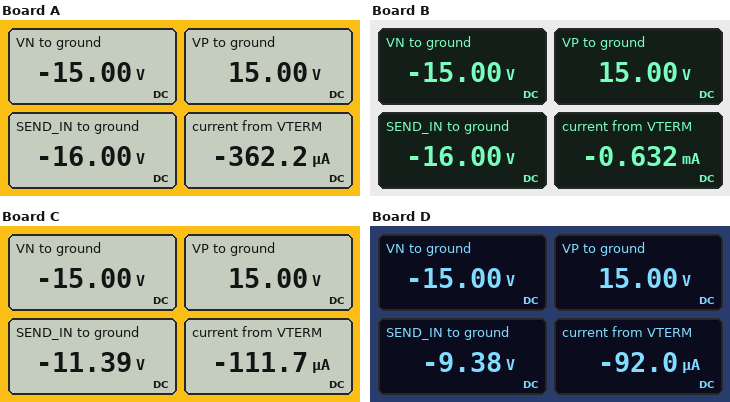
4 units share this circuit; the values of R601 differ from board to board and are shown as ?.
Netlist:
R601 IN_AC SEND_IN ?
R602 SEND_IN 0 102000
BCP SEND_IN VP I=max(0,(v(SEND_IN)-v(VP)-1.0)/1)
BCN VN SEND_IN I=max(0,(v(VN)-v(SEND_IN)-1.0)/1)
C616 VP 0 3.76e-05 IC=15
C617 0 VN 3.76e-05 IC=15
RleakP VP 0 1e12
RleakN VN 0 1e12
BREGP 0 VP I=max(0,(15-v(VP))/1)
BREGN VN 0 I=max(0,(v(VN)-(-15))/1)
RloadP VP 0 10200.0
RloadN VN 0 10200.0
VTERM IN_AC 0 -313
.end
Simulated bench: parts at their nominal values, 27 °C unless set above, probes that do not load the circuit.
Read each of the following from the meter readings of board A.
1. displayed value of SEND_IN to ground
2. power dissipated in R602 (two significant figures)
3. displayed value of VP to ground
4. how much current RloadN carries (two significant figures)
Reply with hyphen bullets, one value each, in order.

- -16.00 V
- 2.5 mW
- 15.00 V
- 1.5 mA
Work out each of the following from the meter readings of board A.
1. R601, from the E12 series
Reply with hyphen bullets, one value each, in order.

- 820 kΩ
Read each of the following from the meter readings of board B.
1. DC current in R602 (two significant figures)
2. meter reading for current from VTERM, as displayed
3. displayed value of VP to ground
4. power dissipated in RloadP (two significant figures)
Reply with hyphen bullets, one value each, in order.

- 160 µA
- -0.632 mA
- 15.00 V
- 22 mW
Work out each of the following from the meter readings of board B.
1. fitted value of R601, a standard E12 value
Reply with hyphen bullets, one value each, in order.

- 470 kΩ
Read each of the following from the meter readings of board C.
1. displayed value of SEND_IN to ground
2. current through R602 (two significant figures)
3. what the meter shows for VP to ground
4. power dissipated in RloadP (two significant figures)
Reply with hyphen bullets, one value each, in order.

- -11.39 V
- 110 µA
- 15.00 V
- 22 mW
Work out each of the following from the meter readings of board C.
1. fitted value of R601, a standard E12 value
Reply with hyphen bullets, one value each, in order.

- 2.7 MΩ
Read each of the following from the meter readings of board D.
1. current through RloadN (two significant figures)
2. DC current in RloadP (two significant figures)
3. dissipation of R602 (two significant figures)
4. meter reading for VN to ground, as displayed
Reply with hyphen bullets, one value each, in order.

- 1.5 mA
- 1.5 mA
- 860 µW
- -15.00 V
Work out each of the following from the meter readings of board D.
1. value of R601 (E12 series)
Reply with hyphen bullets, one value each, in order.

- 3.3 MΩ
